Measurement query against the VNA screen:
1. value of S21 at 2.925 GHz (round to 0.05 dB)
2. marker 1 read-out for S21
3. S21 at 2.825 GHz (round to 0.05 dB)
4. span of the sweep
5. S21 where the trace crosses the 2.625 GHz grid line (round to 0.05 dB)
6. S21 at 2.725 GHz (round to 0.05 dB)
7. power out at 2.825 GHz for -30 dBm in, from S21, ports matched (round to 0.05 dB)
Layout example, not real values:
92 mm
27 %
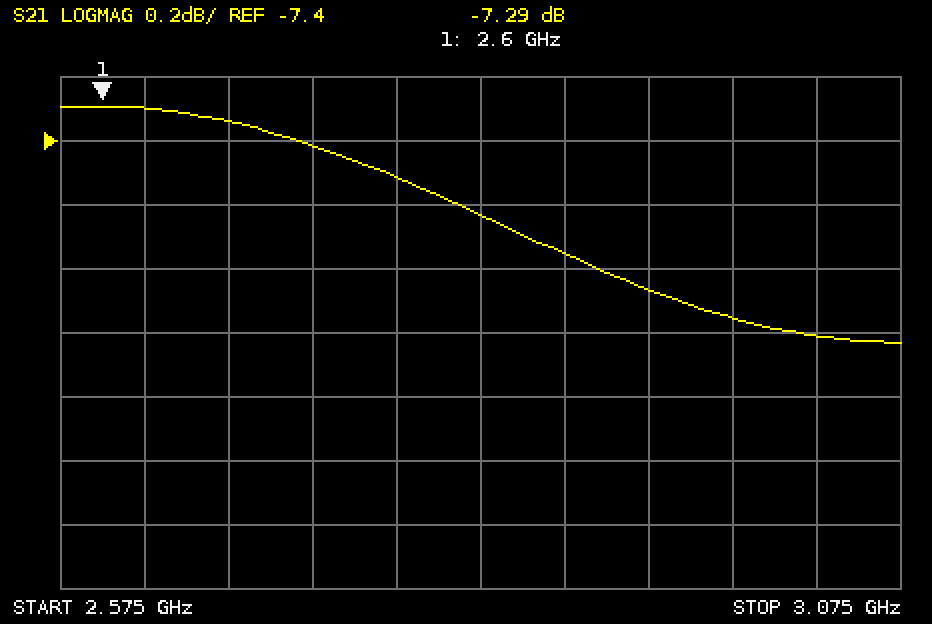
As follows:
-7.85 dB
-7.29 dB
-7.65 dB
500 MHz
-7.30 dB
-7.40 dB
-37.65 dBm
